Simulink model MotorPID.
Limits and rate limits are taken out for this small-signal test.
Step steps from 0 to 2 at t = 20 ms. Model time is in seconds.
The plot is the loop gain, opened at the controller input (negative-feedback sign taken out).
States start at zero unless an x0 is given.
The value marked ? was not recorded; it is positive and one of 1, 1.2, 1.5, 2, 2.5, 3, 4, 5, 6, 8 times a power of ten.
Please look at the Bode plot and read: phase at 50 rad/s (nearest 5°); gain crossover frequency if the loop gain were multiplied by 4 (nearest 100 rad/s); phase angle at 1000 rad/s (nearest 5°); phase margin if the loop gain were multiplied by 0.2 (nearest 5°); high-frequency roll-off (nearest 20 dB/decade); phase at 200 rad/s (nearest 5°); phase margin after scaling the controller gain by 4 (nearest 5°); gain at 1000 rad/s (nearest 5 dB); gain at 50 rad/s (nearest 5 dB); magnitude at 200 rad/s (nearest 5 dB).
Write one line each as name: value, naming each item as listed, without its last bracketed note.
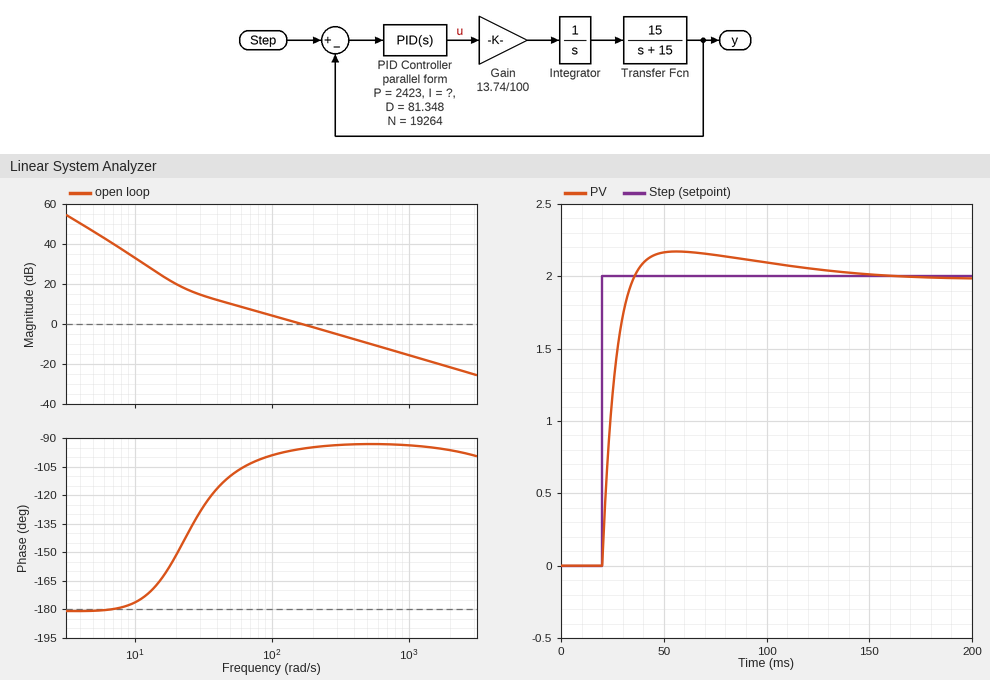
phase at 50 rad/s: -110°
gain crossover frequency if the loop gain were multiplied by 4: 700 rad/s
phase angle at 1000 rad/s: -95°
phase margin if the loop gain were multiplied by 0.2: 55°
high-frequency roll-off: -20 dB/decade
phase at 200 rad/s: -95°
phase margin after scaling the controller gain by 4: 85°
gain at 1000 rad/s: -15 dB
gain at 50 rad/s: 10 dB
magnitude at 200 rad/s: 0 dB
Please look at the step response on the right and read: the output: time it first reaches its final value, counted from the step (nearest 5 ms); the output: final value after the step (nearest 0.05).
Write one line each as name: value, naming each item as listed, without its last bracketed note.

the output: time it first reaches its final value, counted from the step: 15 ms
the output: final value after the step: 2.00
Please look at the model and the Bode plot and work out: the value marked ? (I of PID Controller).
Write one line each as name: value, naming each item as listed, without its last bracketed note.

the value marked ?: 40000
